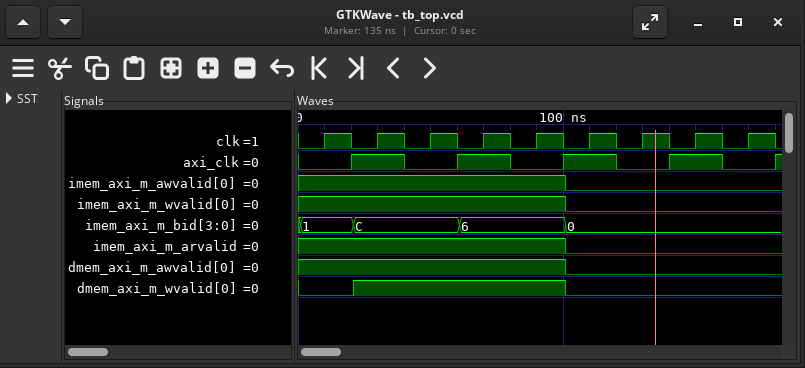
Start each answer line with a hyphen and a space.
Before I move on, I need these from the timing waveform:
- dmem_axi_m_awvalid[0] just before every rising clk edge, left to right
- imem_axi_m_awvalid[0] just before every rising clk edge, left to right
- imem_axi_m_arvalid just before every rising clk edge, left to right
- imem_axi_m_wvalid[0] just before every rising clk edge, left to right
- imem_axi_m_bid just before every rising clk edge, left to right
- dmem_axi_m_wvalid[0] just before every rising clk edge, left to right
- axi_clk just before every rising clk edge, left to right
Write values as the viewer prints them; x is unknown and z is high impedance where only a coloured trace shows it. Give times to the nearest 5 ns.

- 1 1 1 1 1 0 0 0 0
- 1 1 1 1 1 0 0 0 0
- 1 1 1 1 1 0 0 0 0
- 1 1 1 1 1 0 0 0 0
- 1, C, C, 6, 6, 0, 0, 0, 0
- 0 1 1 1 1 0 0 0 0
- 0 1 0 1 0 1 0 1 0
